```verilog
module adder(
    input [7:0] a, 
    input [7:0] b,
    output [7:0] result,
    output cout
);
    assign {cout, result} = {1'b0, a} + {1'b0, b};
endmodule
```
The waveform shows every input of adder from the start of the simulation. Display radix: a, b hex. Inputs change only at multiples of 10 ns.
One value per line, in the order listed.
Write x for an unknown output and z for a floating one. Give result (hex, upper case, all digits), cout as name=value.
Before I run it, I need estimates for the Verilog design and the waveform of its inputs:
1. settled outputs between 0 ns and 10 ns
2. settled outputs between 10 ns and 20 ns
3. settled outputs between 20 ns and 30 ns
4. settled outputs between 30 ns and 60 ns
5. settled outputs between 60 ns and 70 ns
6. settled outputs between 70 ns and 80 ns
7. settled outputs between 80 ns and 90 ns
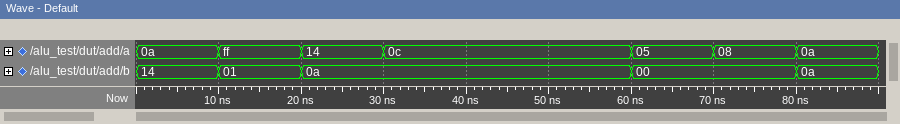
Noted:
result=1E, cout=0
result=00, cout=1
result=1E, cout=0
result=16, cout=0
result=05, cout=0
result=08, cout=0
result=14, cout=0
